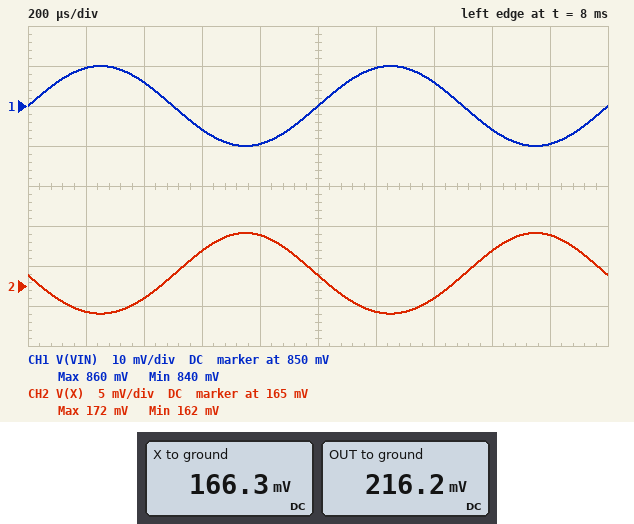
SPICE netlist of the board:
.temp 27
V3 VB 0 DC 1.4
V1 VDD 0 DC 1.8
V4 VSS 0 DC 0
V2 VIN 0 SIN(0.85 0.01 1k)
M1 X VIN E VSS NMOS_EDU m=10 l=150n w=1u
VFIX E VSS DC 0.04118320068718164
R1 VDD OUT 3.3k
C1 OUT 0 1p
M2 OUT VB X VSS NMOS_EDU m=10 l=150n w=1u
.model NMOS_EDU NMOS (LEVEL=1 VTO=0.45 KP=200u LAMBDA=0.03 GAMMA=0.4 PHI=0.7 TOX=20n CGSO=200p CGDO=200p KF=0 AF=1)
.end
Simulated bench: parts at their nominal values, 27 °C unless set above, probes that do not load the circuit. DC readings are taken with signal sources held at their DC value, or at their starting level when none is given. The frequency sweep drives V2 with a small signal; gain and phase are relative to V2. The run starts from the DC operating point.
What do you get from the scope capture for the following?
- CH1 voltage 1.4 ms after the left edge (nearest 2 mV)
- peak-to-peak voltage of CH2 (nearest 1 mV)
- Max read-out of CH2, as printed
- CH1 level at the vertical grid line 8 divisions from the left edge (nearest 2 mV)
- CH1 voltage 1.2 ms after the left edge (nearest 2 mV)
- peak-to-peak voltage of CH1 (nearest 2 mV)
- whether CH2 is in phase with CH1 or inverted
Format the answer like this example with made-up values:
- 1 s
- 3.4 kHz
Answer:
- 856 mV
- 10 mV
- 172 mV
- 844 mV
- 860 mV
- 20 mV
- inverted
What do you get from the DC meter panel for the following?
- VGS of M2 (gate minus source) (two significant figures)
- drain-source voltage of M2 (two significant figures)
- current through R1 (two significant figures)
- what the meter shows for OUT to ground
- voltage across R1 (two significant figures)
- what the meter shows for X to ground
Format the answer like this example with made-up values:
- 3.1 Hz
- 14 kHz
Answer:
- 1.2 V
- 50 mV
- 480 µA
- 216.2 mV
- 1.6 V
- 166.3 mV
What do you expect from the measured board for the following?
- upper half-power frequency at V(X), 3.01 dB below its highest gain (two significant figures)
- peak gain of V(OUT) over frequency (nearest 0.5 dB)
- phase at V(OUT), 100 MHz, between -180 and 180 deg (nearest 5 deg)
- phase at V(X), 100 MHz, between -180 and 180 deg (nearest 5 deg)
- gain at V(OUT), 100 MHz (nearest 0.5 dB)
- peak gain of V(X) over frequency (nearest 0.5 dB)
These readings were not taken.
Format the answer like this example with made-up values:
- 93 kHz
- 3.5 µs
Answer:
- 410 MHz
- -5.5 dB
- 165 deg
- 170 deg
- -6.0 dB
- -6.0 dB
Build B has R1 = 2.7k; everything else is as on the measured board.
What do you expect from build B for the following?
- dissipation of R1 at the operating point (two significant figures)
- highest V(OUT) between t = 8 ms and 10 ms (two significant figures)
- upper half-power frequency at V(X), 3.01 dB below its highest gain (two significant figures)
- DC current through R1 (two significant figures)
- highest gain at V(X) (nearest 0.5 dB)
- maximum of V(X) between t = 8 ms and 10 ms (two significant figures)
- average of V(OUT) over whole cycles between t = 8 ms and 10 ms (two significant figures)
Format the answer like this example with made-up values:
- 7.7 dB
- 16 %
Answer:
- 880 µW
- 270 mV
- 370 MHz
- 570 µA
- -3.0 dB
- 210 mV
- 260 mV
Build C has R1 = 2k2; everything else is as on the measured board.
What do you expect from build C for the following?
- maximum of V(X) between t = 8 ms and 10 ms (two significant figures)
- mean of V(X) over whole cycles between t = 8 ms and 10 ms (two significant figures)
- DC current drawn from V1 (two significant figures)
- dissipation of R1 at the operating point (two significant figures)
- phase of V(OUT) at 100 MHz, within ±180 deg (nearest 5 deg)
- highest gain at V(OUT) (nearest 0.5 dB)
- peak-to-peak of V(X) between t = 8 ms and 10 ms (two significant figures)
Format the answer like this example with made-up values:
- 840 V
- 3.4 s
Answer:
- 250 mV
- 240 mV
- 670 µA
- 990 µW
- 160 deg
- 1.5 dB
- 22 mV
